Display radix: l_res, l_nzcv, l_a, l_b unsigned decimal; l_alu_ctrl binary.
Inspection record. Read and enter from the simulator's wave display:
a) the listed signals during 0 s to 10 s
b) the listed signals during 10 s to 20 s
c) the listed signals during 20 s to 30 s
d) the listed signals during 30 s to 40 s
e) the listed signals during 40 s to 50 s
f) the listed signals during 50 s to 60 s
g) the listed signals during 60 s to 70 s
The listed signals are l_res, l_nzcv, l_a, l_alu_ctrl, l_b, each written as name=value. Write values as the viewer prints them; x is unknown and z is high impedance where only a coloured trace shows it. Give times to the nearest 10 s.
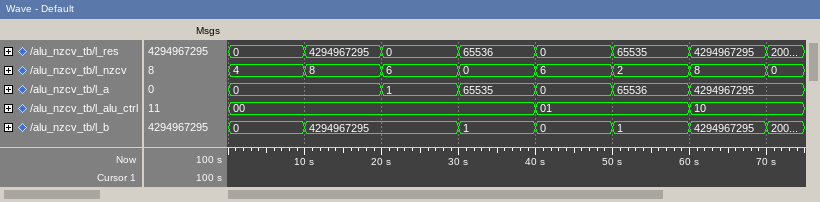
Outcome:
l_res=0, l_nzcv=4, l_a=0, l_alu_ctrl=00, l_b=0
l_res=4294967295, l_nzcv=8, l_a=0, l_alu_ctrl=00, l_b=4294967295
l_res=0, l_nzcv=6, l_a=1, l_alu_ctrl=00, l_b=4294967295
l_res=65536, l_nzcv=0, l_a=65535, l_alu_ctrl=00, l_b=1
l_res=0, l_nzcv=6, l_a=0, l_alu_ctrl=01, l_b=0
l_res=65535, l_nzcv=2, l_a=65536, l_alu_ctrl=01, l_b=1
l_res=4294967295, l_nzcv=8, l_a=4294967295, l_alu_ctrl=10, l_b=4294967295
